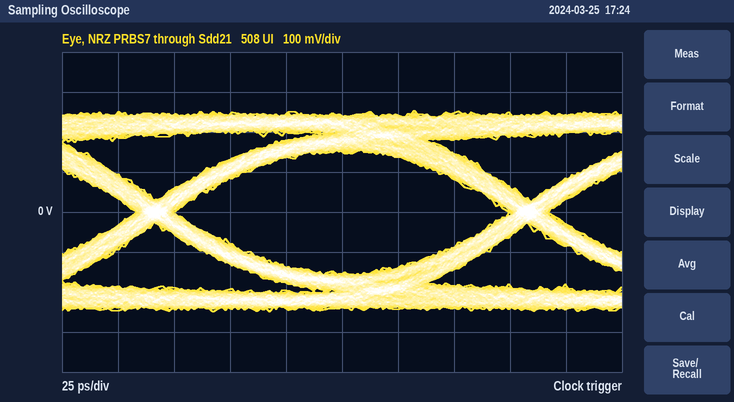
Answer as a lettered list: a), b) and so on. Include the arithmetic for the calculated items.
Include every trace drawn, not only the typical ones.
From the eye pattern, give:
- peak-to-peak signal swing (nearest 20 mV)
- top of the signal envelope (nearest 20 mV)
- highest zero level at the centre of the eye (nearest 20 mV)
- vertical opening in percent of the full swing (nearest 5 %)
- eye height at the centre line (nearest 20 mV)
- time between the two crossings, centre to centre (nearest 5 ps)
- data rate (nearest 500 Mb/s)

a) 500 mV
b) 260 mV
c) -160 mV
d) 300 mV / 500 mV ≈ 60 %
e) 300 mV
f) 165 ps
g) 6.0 Gb/s
